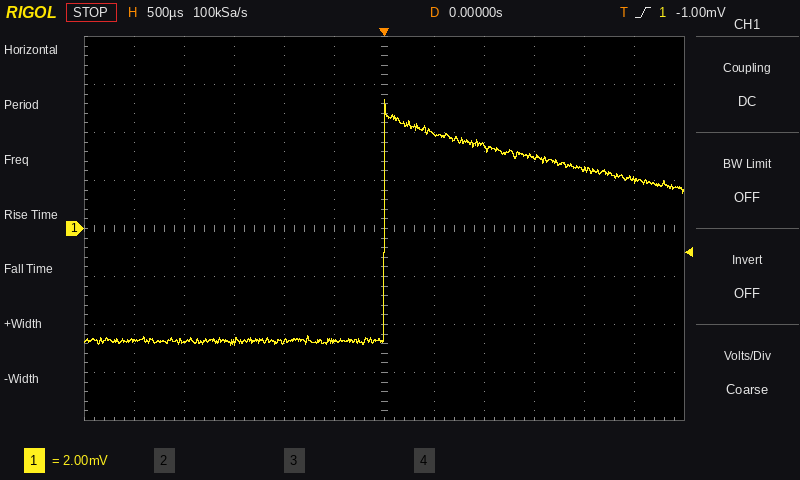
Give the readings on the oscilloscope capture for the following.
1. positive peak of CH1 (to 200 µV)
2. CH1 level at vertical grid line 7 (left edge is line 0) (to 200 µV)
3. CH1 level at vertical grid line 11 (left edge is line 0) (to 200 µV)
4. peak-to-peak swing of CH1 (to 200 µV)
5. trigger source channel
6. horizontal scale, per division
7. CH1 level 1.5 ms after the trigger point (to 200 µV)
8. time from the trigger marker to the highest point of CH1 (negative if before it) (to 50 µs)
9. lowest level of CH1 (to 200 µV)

5.4 mV
4.0 mV
2.0 mV
10.2 mV
CH1
500 µs
3.0 mV
0 µs
-4.8 mV
